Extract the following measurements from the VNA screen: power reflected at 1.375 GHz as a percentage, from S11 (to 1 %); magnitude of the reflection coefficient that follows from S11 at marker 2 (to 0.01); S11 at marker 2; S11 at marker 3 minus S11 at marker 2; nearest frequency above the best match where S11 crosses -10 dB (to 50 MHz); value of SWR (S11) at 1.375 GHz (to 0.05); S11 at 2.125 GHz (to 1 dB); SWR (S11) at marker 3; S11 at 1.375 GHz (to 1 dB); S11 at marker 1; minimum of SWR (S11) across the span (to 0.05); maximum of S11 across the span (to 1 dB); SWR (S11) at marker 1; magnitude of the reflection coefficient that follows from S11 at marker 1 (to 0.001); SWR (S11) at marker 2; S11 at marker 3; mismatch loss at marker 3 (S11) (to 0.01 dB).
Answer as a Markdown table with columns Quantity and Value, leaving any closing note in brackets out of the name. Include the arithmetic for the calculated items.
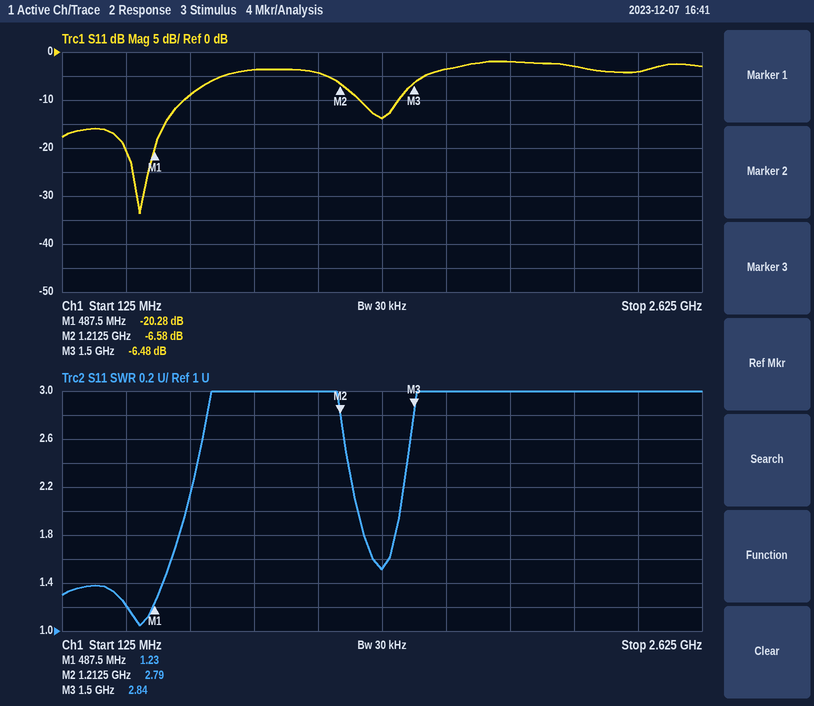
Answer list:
| Quantity | Value |
|---|---|
| power reflected at 1.375 GHz as a percentage, from S11 | 10^(-14/10) ≈ 4 % |
| magnitude of the reflection coefficient that follows from S11 at marker 2 | 10^(-6.58/20) ≈ 0.47 |
| S11 at marker 2 | -6.58 dB |
| S11 at marker 3 minus S11 at marker 2 | -6.48 − (-6.58) = 0.10 dB |
| nearest frequency above the best match where S11 crosses -10 dB | 600 MHz |
| value of SWR (S11) at 1.375 GHz | 1.50 |
| S11 at 2.125 GHz | -3 dB |
| SWR (S11) at marker 3 | 2.84 |
| S11 at 1.375 GHz | -14 dB |
| S11 at marker 1 | -20.28 dB |
| minimum of SWR (S11) across the span | 1.05 |
| maximum of S11 across the span | -2 dB |
| SWR (S11) at marker 1 | 1.23 |
| magnitude of the reflection coefficient that follows from S11 at marker 1 | 10^(-20.28/20) ≈ 0.097 |
| SWR (S11) at marker 2 | 2.79 |
| S11 at marker 3 | -6.48 dB |
| mismatch loss at marker 3 (S11) | −10 log10(1 − 10^(-6.48/10)) ≈ 1.11 dB |
